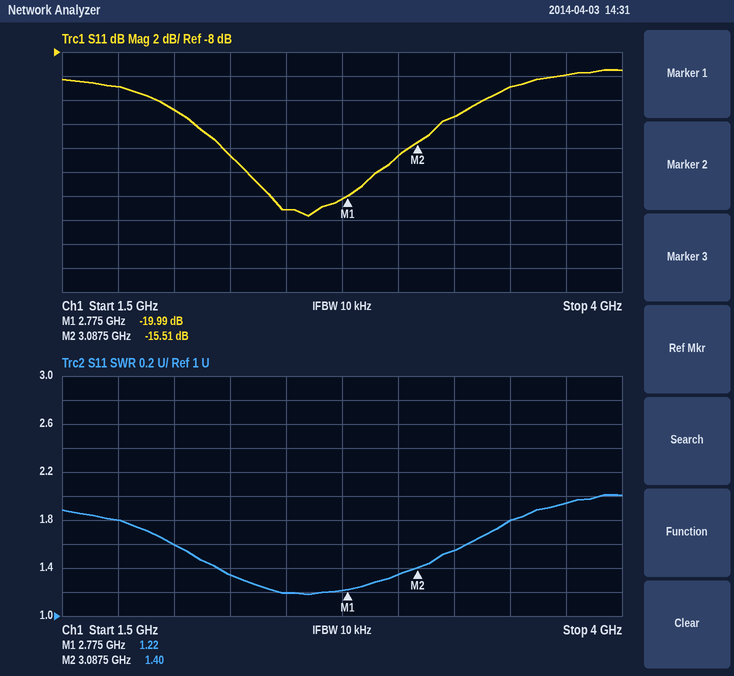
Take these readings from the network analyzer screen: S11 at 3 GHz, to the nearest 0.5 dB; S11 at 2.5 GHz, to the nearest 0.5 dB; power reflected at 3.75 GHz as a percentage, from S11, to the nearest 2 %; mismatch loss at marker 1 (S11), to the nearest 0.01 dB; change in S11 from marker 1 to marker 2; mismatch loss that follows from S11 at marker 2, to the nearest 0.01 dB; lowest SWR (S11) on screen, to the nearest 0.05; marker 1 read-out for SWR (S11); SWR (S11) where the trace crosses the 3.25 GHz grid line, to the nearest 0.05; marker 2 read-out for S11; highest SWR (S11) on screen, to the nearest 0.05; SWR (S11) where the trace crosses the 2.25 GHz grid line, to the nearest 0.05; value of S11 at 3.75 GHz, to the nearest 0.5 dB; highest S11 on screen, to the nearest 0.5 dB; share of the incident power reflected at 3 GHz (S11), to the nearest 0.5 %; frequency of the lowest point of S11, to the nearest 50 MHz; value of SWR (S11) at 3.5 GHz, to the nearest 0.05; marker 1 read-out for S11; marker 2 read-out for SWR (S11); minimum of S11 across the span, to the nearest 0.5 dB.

-16.5 dB
-21.0 dB
10 %
0.04 dB
4.48 dB
0.12 dB
1.20
1.22
1.55
-15.51 dB
2.00
1.35
-10.0 dB
-9.5 dB
2.0 %
2.60 GHz
1.80
-19.99 dB
1.40
-21.5 dB
